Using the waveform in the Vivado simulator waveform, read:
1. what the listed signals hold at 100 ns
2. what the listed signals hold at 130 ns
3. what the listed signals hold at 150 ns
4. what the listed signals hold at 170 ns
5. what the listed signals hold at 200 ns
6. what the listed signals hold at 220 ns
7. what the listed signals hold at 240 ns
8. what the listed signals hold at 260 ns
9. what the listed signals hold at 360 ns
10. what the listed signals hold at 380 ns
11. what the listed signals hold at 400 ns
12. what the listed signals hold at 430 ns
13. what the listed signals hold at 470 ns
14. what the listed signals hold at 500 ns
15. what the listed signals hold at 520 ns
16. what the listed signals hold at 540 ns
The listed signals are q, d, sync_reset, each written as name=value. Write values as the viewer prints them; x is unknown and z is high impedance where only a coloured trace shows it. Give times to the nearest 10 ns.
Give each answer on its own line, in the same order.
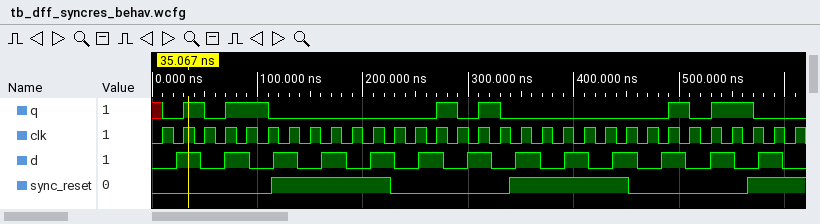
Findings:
q=1, d=0, sync_reset=0
q=0, d=1, sync_reset=1
q=0, d=0, sync_reset=1
q=0, d=1, sync_reset=1
q=0, d=0, sync_reset=1
q=0, d=1, sync_reset=1
q=0, d=0, sync_reset=0
q=0, d=1, sync_reset=0
q=0, d=1, sync_reset=1
q=0, d=0, sync_reset=1
q=0, d=1, sync_reset=1
q=0, d=0, sync_reset=1
q=0, d=0, sync_reset=0
q=1, d=1, sync_reset=0
q=0, d=0, sync_reset=0
q=1, d=1, sync_reset=0
